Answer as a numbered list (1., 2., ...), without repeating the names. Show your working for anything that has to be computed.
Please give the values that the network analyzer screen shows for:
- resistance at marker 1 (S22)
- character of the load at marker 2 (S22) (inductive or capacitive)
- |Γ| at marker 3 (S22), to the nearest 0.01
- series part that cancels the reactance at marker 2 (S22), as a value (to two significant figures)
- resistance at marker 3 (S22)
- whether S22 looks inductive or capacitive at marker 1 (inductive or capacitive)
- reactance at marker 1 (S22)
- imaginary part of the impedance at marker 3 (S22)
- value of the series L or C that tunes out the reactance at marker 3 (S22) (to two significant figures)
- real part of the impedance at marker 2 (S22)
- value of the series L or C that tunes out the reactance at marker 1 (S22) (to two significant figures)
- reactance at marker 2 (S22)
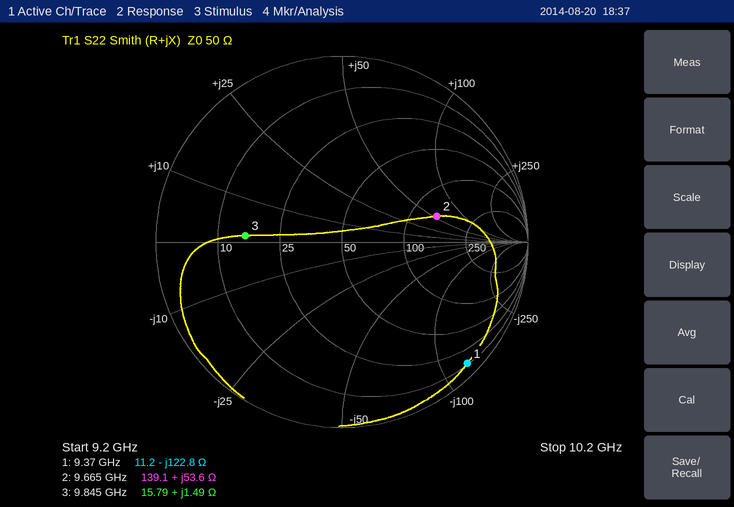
1. 11.2 Ω
2. inductive
3. 0.52
4. C = 1/(2π × 9.665 GHz × 53.6 Ω) ≈ 307 fF, so 310 fF to two significant figures
5. 15.79 Ω
6. capacitive
7. -122.8 Ω
8. +1.49 Ω
9. C = 1/(2π × 9.845 GHz × 1.49 Ω) ≈ 11 pF
10. 139.1 Ω
11. L = 122.8 Ω/(2π × 9.37 GHz) ≈ 2.1 nH
12. +53.6 Ω
